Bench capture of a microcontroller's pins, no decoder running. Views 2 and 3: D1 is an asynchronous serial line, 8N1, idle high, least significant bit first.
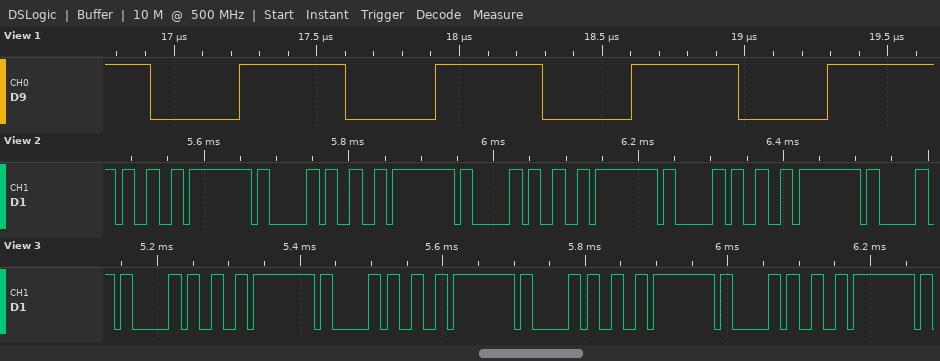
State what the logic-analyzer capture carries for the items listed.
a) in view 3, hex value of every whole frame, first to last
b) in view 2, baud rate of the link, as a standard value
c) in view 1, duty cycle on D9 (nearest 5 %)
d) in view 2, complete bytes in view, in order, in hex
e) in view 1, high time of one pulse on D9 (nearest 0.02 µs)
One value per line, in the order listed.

0x03 0x33 0xFF 0x03 0x33 0xFF 0x03 0x33 0xFF 0x03 0x33 0xFF
115200 baud
55 %
33 FF 03 33 FF 03 33 FF 03 33 FF 03
0.38 µs
